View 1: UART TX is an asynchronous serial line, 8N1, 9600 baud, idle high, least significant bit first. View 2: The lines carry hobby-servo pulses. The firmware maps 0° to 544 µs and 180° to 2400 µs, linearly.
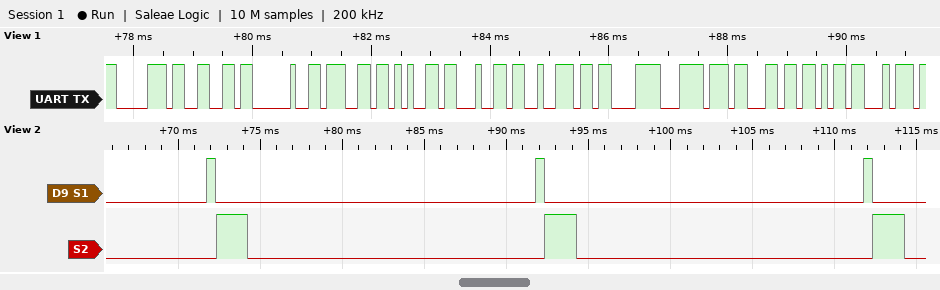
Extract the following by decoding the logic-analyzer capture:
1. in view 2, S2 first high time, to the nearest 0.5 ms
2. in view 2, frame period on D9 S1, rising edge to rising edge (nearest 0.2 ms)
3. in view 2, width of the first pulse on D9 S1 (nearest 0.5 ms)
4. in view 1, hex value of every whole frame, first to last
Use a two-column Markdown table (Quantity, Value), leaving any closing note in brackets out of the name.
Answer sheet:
| Quantity | Value |
|---|---|
| in view 2, S2 first high time, to the nearest 0.5 ms | 2.0 ms |
| in view 2, frame period on D9 S1, rising edge to rising edge | 20.0 ms |
| in view 2, width of the first pulse on D9 S1 | 0.5 ms |
| in view 1, hex value of every whole frame, first to last | 70 66 20 67 65 64 72 C3 BC 63 6B 74 |
